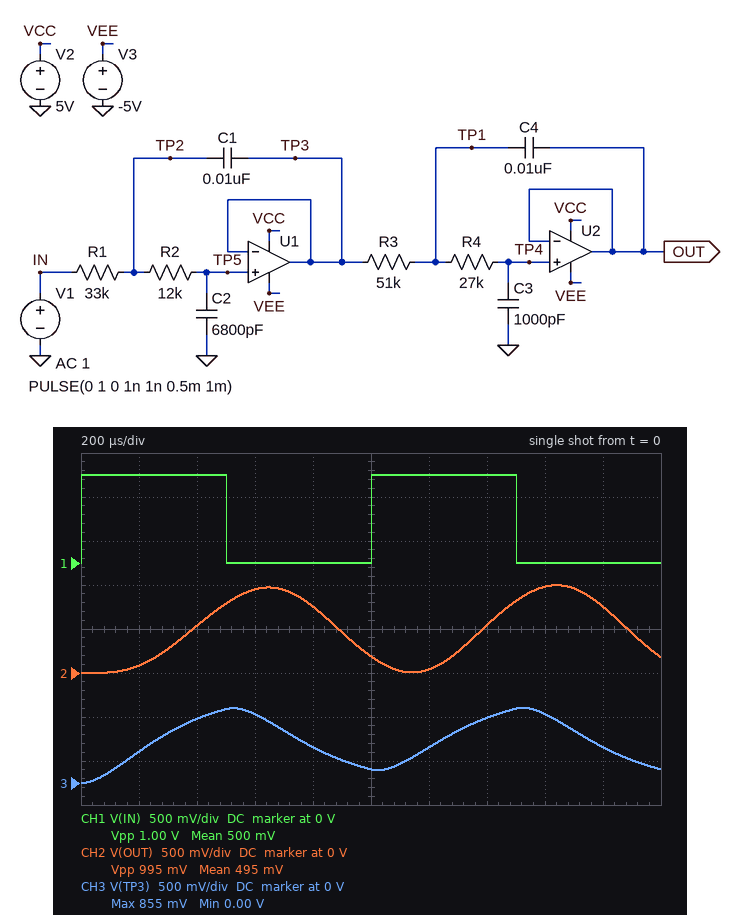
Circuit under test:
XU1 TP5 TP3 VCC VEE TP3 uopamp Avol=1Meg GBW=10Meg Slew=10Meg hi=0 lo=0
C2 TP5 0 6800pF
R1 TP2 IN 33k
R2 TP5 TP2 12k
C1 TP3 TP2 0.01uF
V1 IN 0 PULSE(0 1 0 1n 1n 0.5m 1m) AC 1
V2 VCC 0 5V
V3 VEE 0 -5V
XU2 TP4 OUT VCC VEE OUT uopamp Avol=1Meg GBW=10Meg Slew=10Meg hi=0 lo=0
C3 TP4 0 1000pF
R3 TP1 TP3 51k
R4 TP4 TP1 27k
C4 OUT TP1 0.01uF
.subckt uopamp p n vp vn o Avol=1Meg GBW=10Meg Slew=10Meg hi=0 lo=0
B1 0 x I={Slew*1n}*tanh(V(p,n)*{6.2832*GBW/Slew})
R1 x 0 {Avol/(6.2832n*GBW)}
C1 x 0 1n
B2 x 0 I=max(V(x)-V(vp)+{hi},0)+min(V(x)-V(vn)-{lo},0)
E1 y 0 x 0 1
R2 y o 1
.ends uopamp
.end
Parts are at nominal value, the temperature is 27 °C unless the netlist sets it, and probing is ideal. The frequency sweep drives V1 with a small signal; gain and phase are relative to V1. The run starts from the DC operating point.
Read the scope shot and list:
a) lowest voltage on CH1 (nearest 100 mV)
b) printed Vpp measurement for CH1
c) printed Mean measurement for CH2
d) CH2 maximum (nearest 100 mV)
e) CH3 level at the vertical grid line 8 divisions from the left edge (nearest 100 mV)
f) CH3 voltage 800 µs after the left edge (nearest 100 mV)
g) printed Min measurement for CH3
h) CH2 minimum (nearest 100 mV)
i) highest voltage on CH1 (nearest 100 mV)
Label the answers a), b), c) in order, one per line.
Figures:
a) 0 V
b) 1.00 V
c) 495 mV
d) 1.0 V
e) 800 mV
f) 400 mV
g) 0.00 V
h) 0 V
i) 1.0 V
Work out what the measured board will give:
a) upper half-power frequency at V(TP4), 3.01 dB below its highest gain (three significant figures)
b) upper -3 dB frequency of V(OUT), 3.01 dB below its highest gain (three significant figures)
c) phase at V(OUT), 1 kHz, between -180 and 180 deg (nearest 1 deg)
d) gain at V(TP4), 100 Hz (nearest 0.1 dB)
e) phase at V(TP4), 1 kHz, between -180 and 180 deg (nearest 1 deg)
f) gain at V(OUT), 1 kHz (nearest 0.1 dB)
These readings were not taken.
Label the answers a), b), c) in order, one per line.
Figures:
a) 1.15 kHz
b) 1.15 kHz
c) -139 deg
d) 0 dB
e) -139 deg
f) -2.2 dB
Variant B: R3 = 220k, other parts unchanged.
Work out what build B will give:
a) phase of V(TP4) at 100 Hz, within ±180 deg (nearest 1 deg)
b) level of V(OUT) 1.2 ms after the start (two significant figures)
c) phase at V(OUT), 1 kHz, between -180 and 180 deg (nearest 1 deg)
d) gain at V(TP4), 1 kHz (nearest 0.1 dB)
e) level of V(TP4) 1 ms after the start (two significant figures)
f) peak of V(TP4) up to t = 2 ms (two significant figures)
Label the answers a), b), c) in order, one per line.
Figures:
a) -20 deg
b) 460 mV
c) 137 deg
d) -11.9 dB
e) 680 mV
f) 740 mV
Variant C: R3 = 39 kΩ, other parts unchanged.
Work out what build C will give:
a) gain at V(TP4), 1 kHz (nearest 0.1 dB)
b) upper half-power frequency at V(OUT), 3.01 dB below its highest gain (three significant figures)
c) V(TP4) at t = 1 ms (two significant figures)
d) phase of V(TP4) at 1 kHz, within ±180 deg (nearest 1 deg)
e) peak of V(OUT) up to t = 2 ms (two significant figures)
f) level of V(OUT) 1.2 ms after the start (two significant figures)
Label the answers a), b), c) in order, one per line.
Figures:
a) -2.8 dB
b) 1.06 kHz
c) 140 mV
d) -127 deg
e) 960 mV
f) 110 mV
